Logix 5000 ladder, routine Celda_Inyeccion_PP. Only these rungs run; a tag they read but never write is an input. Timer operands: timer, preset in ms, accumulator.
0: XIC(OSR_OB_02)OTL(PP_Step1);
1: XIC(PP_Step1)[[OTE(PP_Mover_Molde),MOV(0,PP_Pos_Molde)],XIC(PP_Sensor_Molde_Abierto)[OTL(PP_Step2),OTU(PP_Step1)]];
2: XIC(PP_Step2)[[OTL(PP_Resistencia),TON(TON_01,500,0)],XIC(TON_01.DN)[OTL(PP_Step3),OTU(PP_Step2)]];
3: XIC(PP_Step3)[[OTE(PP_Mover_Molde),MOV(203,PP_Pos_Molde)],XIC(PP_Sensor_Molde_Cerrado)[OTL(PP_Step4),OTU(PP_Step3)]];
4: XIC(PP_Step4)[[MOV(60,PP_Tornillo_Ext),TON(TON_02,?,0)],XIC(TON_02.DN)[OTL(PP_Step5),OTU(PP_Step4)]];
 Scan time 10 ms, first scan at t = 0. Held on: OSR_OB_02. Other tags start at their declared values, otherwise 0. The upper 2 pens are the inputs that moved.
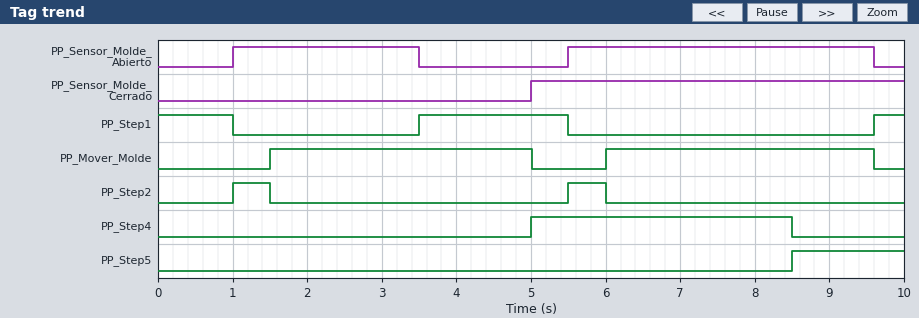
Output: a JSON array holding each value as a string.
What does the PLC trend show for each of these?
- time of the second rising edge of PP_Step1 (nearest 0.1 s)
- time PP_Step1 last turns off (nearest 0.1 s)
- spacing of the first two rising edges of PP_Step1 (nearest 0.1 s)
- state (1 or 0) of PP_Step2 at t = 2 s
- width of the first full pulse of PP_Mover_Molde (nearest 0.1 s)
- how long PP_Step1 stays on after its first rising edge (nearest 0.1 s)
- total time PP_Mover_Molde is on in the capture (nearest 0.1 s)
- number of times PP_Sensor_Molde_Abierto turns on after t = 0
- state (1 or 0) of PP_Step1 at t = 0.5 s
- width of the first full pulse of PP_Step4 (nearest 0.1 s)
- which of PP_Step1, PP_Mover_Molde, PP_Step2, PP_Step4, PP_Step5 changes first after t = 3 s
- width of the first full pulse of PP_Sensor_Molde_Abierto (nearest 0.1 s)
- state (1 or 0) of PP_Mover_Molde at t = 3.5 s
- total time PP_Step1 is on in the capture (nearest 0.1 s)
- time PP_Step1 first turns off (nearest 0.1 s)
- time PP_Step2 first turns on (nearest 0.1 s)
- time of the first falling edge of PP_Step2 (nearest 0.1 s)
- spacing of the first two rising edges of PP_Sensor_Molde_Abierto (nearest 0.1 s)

["9.6 s", "5.5 s", "6.1 s", "0", "3.5 s", "2.0 s", "7.1 s", "2", "1", "3.5 s", "PP_Step1", "2.5 s", "1", "3.4 s", "1.0 s", "1.0 s", "1.5 s", "4.5 s"]
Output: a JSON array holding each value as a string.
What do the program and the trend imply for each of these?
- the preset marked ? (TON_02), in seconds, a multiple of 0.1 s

["3.5 s"]
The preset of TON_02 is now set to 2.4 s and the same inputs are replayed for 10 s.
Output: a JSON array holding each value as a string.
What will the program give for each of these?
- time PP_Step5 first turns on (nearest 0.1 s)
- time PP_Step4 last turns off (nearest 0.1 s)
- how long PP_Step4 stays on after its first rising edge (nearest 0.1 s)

["7.4 s", "7.4 s", "2.4 s"]
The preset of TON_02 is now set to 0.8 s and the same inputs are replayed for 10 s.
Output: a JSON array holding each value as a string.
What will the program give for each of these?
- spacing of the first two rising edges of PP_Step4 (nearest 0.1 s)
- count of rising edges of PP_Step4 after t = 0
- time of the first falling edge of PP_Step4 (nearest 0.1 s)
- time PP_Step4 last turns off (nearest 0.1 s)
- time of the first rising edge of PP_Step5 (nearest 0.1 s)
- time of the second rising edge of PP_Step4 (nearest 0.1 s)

["1.0 s", "2", "5.8 s", "6.8 s", "5.8 s", "6.0 s"]
